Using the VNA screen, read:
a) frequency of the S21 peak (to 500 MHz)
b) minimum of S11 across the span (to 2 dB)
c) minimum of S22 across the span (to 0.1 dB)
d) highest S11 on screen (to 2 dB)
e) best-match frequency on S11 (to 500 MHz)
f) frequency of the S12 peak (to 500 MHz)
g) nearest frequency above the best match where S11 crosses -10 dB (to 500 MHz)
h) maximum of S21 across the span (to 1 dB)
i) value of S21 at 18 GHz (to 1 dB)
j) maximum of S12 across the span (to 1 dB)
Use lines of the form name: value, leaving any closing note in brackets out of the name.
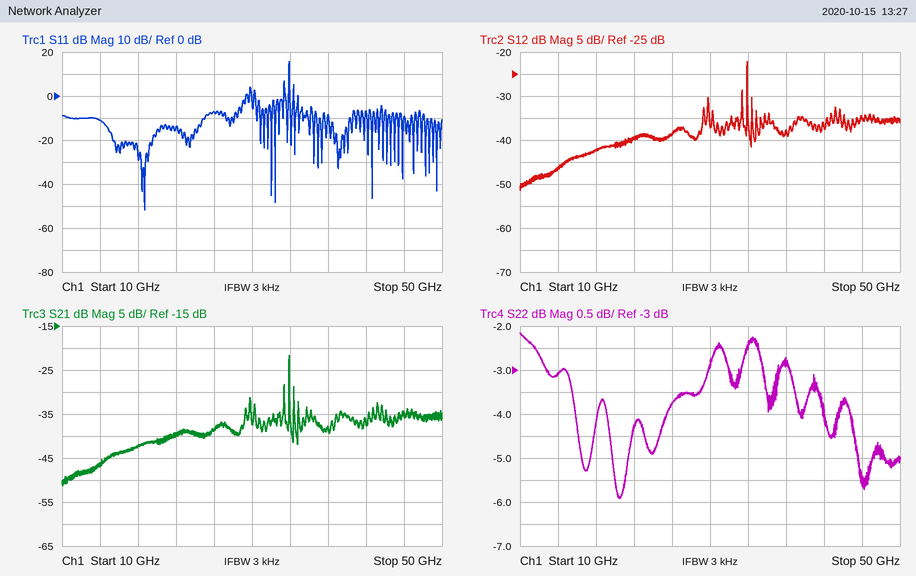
frequency of the S21 peak: 34.0 GHz
minimum of S11 across the span: -52 dB
minimum of S22 across the span: -5.9 dB
highest S11 on screen: 16 dB
best-match frequency on S11: 18.5 GHz
frequency of the S12 peak: 34.0 GHz
nearest frequency above the best match where S11 crosses -10 dB: 25.0 GHz
maximum of S21 across the span: -22 dB
value of S21 at 18 GHz: -42 dB
maximum of S12 across the span: -22 dB
